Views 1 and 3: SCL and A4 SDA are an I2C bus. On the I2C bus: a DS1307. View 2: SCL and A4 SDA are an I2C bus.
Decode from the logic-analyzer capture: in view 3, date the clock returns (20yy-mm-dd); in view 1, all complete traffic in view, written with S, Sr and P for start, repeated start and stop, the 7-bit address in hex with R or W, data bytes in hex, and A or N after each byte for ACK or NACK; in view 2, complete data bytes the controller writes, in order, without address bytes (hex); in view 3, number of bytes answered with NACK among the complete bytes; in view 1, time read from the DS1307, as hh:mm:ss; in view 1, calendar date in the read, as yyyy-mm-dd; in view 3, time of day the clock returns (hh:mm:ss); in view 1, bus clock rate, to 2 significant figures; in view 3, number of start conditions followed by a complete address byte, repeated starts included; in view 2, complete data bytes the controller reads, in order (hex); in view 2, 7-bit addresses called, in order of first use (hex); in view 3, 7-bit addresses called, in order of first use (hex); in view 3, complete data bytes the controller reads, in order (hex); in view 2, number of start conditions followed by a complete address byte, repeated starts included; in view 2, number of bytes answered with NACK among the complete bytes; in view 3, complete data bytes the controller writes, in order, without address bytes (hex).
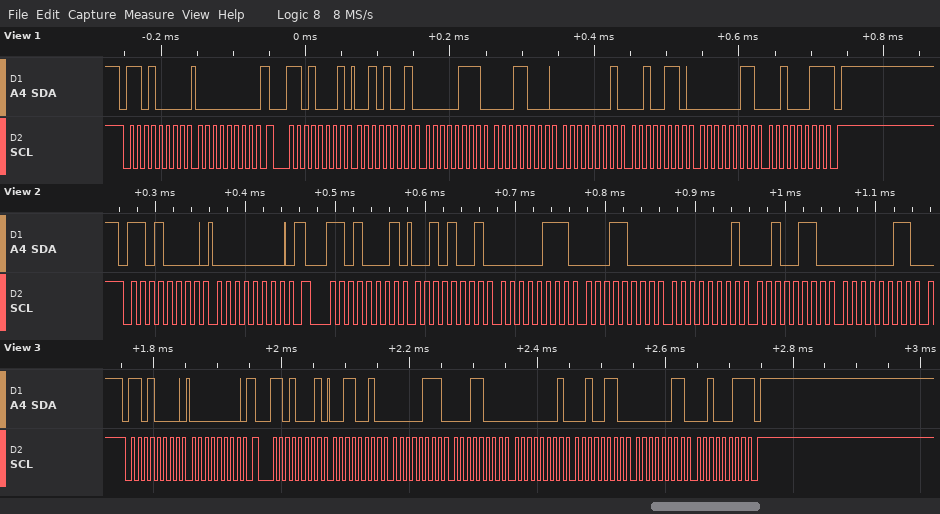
2023-03-26
S 68W A 00 A Sr 68R A 29 A 07 A 18 A 01 A 26 A 03 A 23 N P
00
1
18:07:29
2023-03-26
18:07:32
100 kHz
2
29 07 18 01 26 03
0x68
0x68
32 07 18 01 26 03 23
2
0
00
